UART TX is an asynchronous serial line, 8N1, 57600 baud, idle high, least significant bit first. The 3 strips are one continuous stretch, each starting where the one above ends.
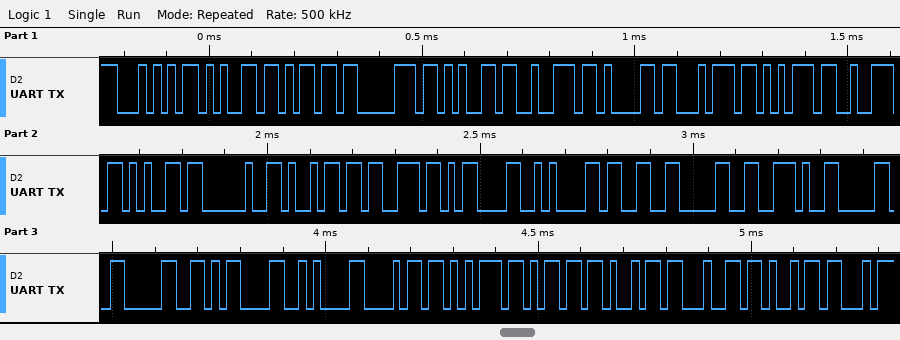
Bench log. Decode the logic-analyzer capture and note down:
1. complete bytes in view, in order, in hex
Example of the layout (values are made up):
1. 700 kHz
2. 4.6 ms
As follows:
1. 54 65 6D 70 65 72 61 74 75 72 65 20 69 73 0D 0A 33 30 2E 30 30 0D 0A 68 75 6D 69 64 69
